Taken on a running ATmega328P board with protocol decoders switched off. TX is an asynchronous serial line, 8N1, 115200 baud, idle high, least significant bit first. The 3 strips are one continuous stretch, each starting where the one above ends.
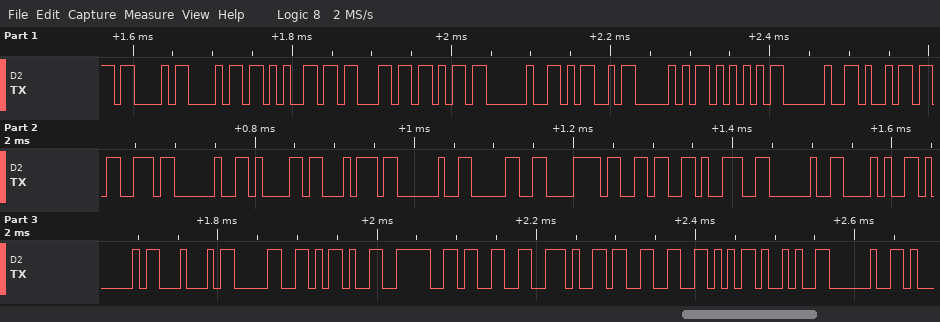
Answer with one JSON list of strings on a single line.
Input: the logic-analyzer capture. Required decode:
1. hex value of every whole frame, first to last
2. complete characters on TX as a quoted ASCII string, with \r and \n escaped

["43 68 65 63 6B 20 4D 50 55 20 69 73 20 61 74 20 30 78 36 39 20 28 41 44 30 2D 3E 33 2E 33 56 29 20", "\"Check MPU is at 0x69 (AD0->3.3V) \""]
